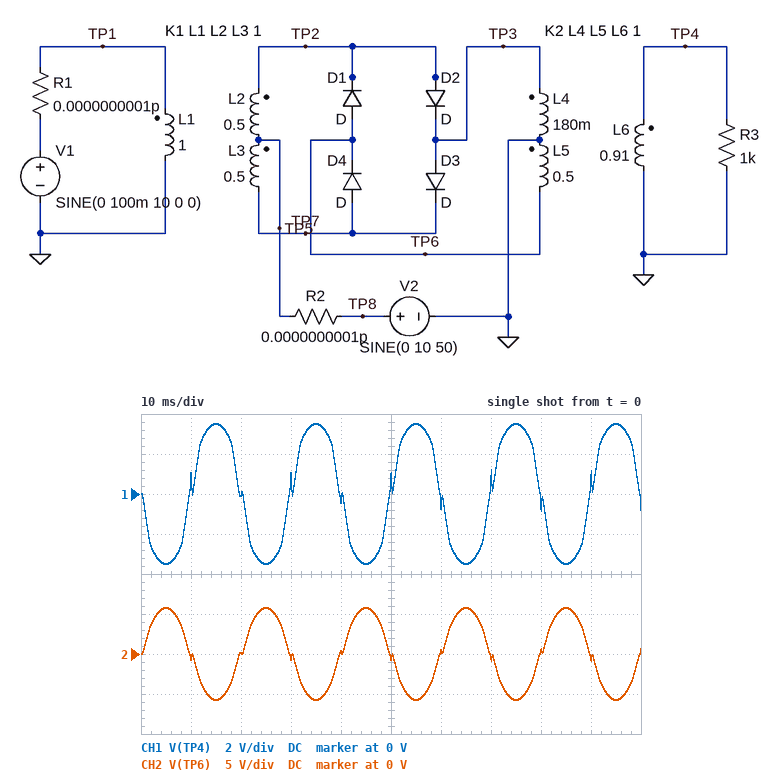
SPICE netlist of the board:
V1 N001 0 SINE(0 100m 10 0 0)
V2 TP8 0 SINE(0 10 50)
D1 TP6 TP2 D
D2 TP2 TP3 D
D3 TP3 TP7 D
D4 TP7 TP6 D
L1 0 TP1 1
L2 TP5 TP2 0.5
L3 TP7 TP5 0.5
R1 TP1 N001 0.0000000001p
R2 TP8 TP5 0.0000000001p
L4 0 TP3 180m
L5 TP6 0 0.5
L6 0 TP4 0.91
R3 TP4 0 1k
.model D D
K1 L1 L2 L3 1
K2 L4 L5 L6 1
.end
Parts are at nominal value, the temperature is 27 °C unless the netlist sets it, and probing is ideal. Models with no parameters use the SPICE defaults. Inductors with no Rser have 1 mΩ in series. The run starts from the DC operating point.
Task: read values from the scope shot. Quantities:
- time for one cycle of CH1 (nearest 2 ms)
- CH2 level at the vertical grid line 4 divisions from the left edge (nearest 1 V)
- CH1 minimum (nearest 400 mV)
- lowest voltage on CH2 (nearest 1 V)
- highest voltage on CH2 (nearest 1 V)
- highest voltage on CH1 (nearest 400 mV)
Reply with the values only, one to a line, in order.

20 ms
0 V
-3.6 V
-6 V
6 V
3.6 V
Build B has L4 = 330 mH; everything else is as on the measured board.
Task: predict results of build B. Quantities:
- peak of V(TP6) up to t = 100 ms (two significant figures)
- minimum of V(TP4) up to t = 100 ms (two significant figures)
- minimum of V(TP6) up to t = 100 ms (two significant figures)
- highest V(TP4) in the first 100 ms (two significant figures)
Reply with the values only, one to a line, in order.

5.5 V
-2.1 V
-5.5 V
2.1 V
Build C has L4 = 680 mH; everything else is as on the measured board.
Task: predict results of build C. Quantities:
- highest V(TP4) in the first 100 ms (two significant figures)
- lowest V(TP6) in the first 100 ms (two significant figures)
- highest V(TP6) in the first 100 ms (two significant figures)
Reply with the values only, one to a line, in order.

1.4 V
-3.9 V
3.9 V
